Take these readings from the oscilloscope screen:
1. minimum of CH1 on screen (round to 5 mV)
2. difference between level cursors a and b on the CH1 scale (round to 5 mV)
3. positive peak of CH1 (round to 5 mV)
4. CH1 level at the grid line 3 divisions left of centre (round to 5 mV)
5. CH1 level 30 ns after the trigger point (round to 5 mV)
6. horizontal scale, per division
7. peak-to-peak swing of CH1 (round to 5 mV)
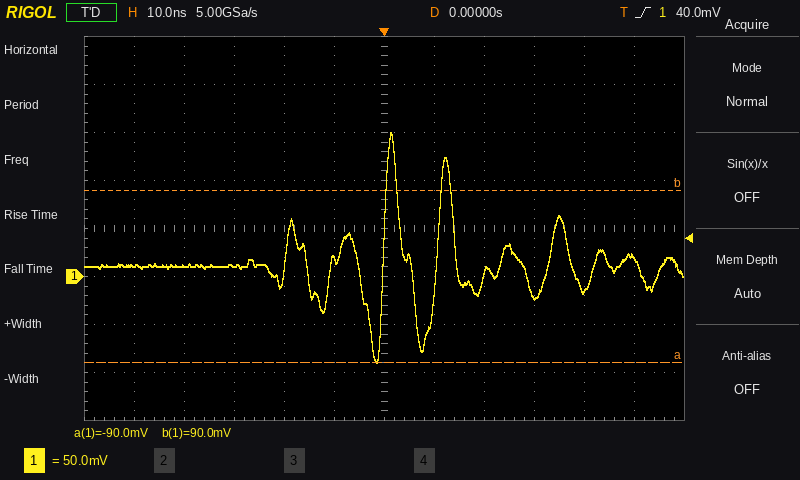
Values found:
-90 mV
180 mV
150 mV
10 mV
-20 mV
10 ns
240 mV
